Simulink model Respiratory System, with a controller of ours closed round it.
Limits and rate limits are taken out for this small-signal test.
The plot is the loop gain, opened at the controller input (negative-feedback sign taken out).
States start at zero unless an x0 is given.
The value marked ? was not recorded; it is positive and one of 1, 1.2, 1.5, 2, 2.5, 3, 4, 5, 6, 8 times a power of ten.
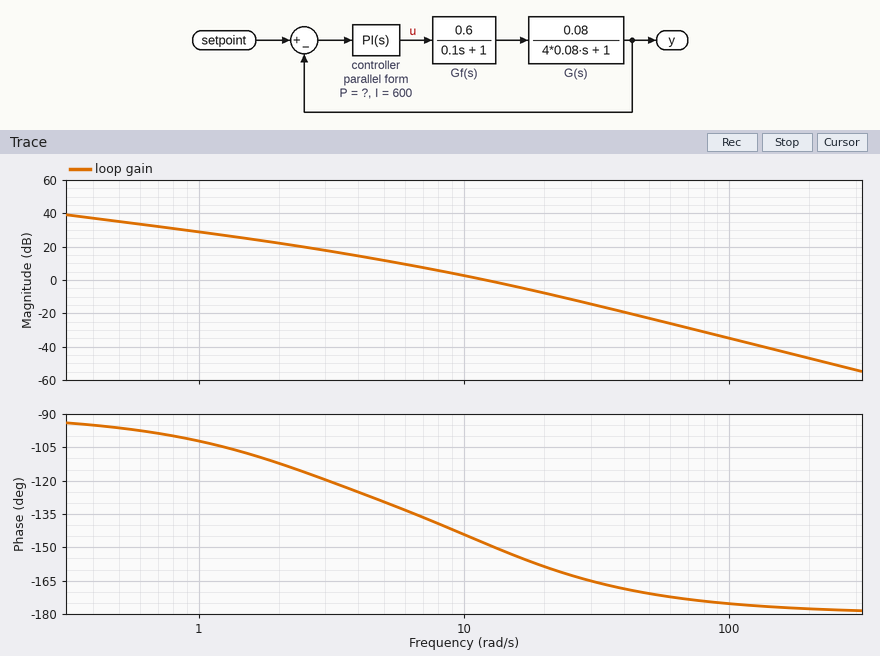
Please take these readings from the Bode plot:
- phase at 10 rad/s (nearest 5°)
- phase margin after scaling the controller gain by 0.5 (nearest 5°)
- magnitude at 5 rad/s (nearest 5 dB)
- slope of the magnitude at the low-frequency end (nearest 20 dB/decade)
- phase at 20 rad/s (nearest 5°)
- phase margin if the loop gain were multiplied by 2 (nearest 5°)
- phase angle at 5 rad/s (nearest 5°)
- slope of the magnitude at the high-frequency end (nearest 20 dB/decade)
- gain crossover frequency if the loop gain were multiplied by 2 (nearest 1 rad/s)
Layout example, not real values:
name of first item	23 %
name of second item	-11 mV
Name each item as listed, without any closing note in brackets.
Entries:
phase at 10 rad/s	-145°
phase margin after scaling the controller gain by 0.5	40°
magnitude at 5 rad/s	10 dB
slope of the magnitude at the low-frequency end	-20 dB/decade
phase at 20 rad/s	-160°
phase margin if the loop gain were multiplied by 2	25°
phase angle at 5 rad/s	-130°
slope of the magnitude at the high-frequency end	-40 dB/decade
gain crossover frequency if the loop gain were multiplied by 2	18 rad/s
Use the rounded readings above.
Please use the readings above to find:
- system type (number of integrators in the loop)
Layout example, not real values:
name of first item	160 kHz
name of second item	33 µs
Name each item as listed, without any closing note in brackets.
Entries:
system type	1
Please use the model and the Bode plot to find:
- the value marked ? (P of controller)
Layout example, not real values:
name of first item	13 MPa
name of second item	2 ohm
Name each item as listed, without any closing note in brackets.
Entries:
the value marked ?	120
